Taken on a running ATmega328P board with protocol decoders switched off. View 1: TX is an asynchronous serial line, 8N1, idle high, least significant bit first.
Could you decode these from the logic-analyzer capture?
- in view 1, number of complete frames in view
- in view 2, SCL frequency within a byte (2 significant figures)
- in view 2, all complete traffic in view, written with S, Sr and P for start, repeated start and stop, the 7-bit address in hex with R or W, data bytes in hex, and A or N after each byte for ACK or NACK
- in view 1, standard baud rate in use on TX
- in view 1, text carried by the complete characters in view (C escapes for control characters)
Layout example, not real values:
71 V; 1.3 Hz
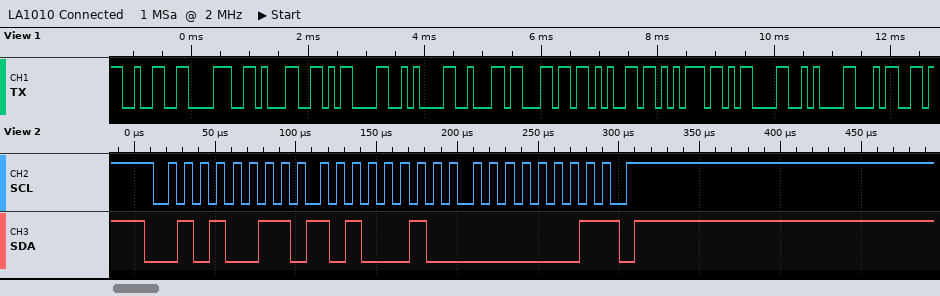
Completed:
12; 100 kHz; S 29R A A2 A 01 N P; 9600 baud; "281\r\nbleu\r\n4"
